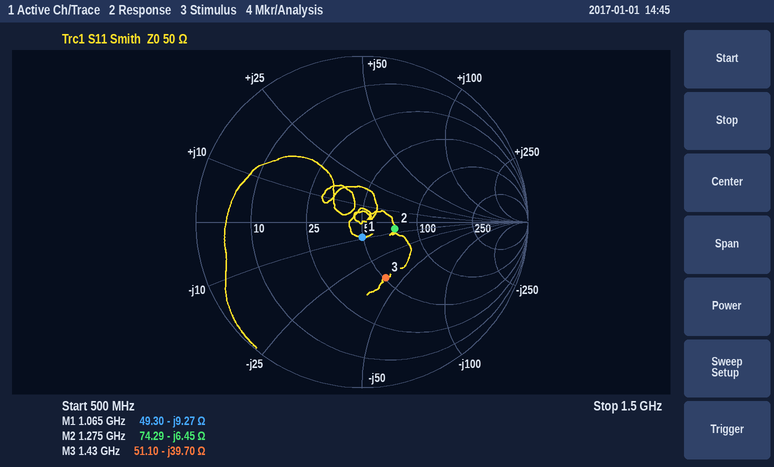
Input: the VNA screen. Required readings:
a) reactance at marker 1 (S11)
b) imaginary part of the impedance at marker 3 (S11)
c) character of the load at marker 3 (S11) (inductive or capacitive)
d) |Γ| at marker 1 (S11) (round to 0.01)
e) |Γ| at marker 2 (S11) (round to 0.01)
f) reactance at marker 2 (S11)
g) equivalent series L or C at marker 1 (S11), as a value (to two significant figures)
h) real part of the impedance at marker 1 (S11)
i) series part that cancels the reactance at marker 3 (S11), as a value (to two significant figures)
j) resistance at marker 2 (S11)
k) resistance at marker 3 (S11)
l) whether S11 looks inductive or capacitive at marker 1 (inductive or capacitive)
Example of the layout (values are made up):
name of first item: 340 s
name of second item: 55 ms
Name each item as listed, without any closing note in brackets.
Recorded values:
reactance at marker 1: -9.27 Ω
imaginary part of the impedance at marker 3: -39.70 Ω
character of the load at marker 3 (S11): capacitive
|Γ| at marker 1 (S11): 0.09
|Γ| at marker 2 (S11): 0.20
reactance at marker 2: -6.45 Ω
equivalent series L or C at marker 1 (S11), as a value: 16 pF
real part of the impedance at marker 1: 49.30 Ω
series part that cancels the reactance at marker 3 (S11), as a value: 4.4 nH
resistance at marker 2: 74.29 Ω
resistance at marker 3: 51.10 Ω
whether S11 looks inductive or capacitive at marker 1: capacitive
